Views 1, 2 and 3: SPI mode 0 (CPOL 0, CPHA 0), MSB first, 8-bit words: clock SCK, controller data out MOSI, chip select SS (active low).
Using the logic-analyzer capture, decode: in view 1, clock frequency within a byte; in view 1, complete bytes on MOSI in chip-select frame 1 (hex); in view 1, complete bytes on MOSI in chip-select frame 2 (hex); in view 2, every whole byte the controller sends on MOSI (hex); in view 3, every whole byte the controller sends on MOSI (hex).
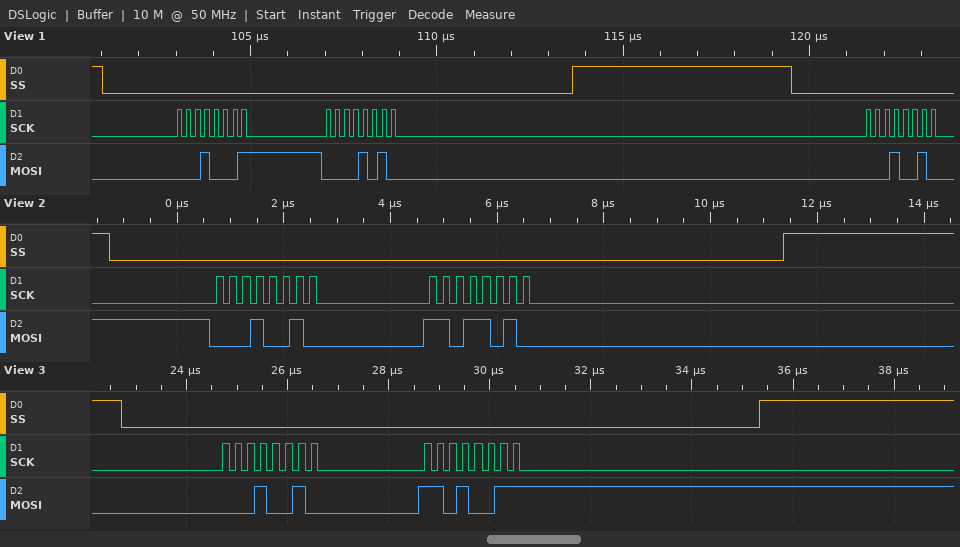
4 MHz
11 0A
12
12 DA
0x12 0xD3
